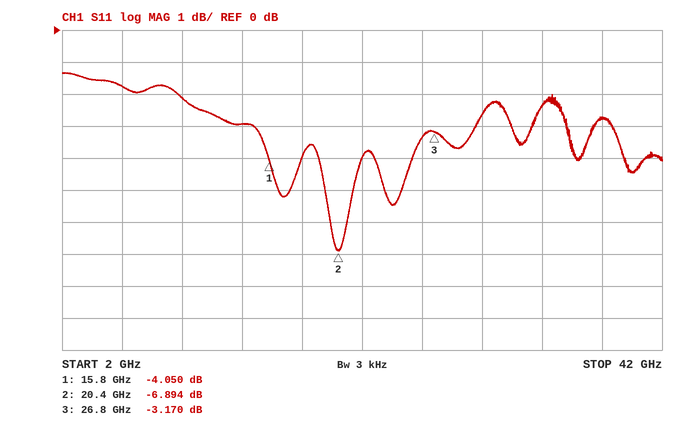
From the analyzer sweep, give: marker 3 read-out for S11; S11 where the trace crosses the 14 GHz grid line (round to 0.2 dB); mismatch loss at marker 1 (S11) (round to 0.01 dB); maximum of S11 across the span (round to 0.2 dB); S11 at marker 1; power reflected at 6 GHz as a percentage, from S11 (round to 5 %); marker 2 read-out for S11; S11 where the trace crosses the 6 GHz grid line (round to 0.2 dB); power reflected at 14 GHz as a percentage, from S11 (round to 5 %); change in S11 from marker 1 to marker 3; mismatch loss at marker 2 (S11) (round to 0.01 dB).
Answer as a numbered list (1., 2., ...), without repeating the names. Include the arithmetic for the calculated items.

1. -3.170 dB
2. -3.0 dB
3. −10 log10(1 − 10^(-4.05/10)) ≈ 2.17 dB
4. -1.4 dB
5. -4.050 dB
6. 10^(-1.8/10) ≈ 66.1 %, so 65 % to the nearest 5 %
7. -6.894 dB
8. -1.8 dB
9. 10^(-3/10) ≈ 50 %
10. -3.17 − (-4.05) = 0.880 dB
11. −10 log10(1 − 10^(-6.894/10)) ≈ 0.99 dB
